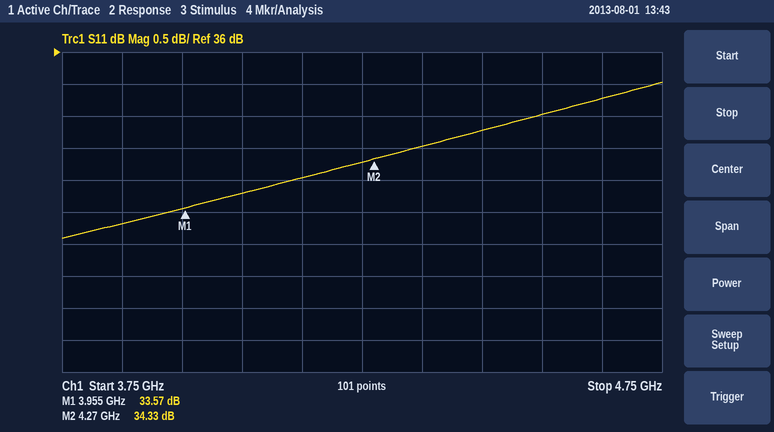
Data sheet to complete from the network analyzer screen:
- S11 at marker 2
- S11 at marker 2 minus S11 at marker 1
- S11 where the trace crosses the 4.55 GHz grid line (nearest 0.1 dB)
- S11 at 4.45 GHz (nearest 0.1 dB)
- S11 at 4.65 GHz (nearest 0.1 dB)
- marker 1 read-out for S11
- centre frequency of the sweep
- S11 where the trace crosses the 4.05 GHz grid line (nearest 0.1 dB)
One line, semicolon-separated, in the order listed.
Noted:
34.33 dB; 0.76 dB; 35.0 dB; 34.8 dB; 35.3 dB; 33.57 dB; 4.25 GHz; 33.8 dB
